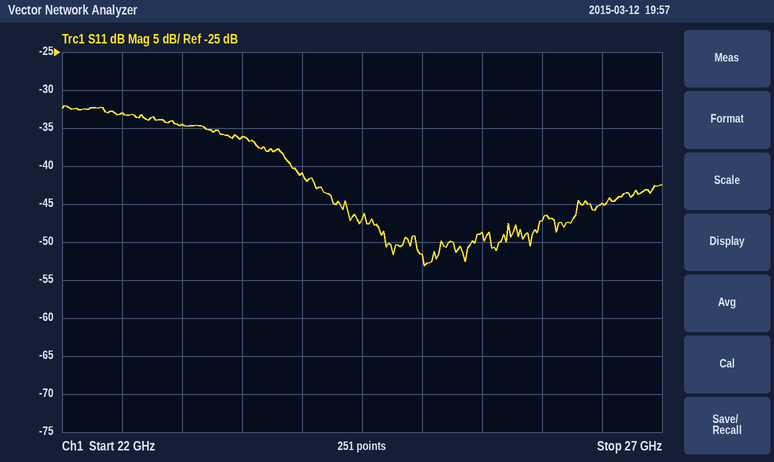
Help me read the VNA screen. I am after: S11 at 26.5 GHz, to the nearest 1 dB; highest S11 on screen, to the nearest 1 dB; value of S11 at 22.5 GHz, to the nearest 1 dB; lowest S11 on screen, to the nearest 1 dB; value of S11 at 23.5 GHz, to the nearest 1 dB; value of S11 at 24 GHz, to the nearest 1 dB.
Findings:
-45 dB
-32 dB
-33 dB
-53 dB
-36 dB
-41 dB
